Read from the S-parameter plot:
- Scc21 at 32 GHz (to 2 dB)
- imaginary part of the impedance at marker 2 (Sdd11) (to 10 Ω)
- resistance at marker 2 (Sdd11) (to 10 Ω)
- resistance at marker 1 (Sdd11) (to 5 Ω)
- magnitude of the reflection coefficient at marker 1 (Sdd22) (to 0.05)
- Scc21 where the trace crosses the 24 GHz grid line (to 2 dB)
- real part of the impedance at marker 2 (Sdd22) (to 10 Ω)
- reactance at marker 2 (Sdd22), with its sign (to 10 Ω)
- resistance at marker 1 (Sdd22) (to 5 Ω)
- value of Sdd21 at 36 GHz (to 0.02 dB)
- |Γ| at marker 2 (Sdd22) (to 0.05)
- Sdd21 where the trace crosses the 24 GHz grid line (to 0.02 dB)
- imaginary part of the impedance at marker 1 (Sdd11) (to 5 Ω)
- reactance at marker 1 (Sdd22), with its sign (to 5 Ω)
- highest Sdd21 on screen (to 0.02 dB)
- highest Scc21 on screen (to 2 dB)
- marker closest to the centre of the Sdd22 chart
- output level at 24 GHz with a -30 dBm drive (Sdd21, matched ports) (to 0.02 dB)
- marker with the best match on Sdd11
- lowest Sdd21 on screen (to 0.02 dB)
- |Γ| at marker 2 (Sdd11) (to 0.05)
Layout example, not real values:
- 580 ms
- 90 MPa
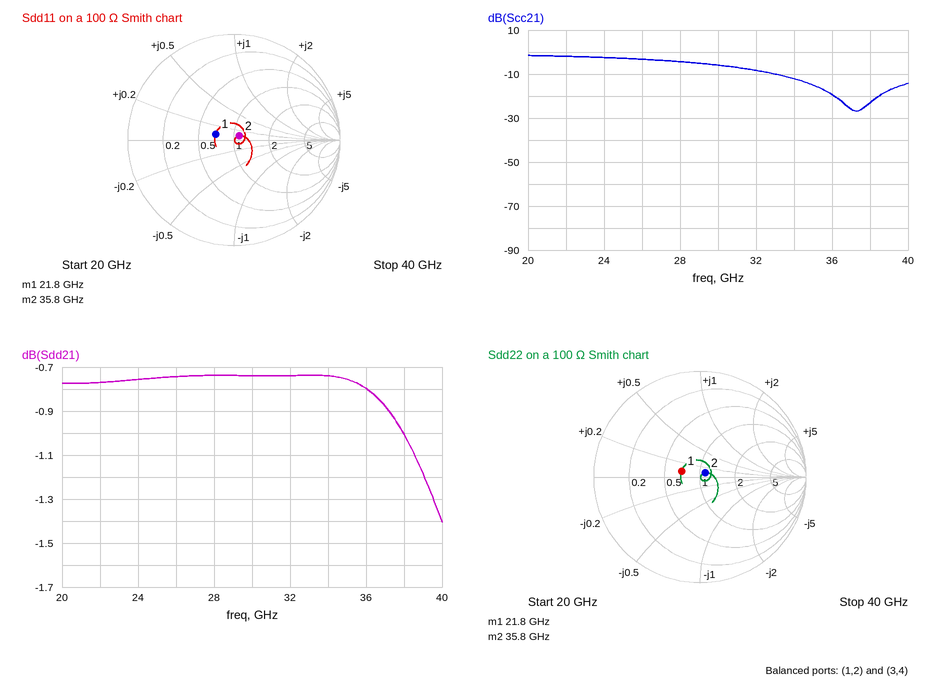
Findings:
- -8 dB
- +10 Ω
- 110 Ω
- 70 Ω
- 0.20
- -2 dB
- 110 Ω
- +10 Ω
- 70 Ω
- -0.80 dB
- 0.05
- -0.76 dB
- +10 Ω
- +10 Ω
- -0.74 dB
- -2 dB
- marker 2
- -30.76 dBm
- marker 2
- -1.40 dB
- 0.05
